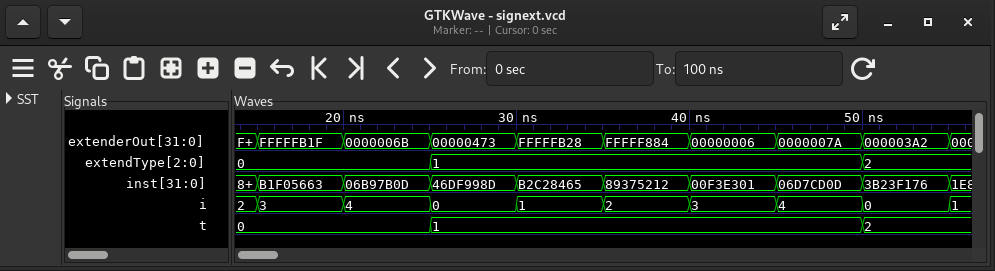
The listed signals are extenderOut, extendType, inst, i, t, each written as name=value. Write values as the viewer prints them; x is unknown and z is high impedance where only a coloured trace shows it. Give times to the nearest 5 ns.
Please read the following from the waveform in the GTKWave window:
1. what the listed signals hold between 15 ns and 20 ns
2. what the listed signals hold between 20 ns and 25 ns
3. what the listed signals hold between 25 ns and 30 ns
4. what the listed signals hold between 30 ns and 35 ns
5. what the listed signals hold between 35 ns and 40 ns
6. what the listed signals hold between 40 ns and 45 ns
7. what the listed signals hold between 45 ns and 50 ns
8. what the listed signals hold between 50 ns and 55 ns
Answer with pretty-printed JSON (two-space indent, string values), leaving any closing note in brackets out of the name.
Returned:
{
  "what the listed signals hold between 15 ns and 20 ns": "extenderOut=FFFFFB1F, extendType=0, inst=B1F05663, i=3, t=0",
  "what the listed signals hold between 20 ns and 25 ns": "extenderOut=0000006B, extendType=0, inst=06B97B0D, i=4, t=0",
  "what the listed signals hold between 25 ns and 30 ns": "extenderOut=00000473, extendType=1, inst=46DF998D, i=0, t=1",
  "what the listed signals hold between 30 ns and 35 ns": "extenderOut=FFFFFB28, extendType=1, inst=B2C28465, i=1, t=1",
  "what the listed signals hold between 35 ns and 40 ns": "extenderOut=FFFFF884, extendType=1, inst=89375212, i=2, t=1",
  "what the listed signals hold between 40 ns and 45 ns": "extenderOut=00000006, extendType=1, inst=00F3E301, i=3, t=1",
  "what the listed signals hold between 45 ns and 50 ns": "extenderOut=0000007A, extendType=1, inst=06D7CD0D, i=4, t=1",
  "what the listed signals hold between 50 ns and 55 ns": "extenderOut=000003A2, extendType=2, inst=3B23F176, i=0, t=2"
}
